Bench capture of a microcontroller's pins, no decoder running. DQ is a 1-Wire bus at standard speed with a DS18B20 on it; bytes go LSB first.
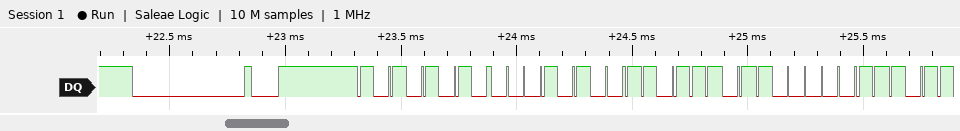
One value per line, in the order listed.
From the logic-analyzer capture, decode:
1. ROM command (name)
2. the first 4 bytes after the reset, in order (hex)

Match ROM
55 28 BB C1
